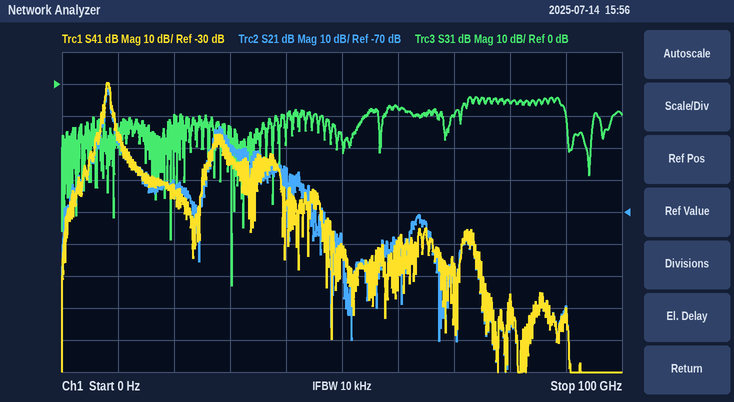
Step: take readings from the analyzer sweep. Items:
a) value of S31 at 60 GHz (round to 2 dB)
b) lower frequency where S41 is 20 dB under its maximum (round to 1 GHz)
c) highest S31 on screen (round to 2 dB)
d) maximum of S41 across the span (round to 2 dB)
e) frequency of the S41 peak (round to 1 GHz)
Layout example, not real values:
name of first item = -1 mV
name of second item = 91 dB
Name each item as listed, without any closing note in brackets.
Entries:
value of S31 at 60 GHz = -8 dB
lower frequency where S41 is 20 dB under its maximum = 6 GHz
highest S31 on screen = -4 dB
maximum of S41 across the span = -30 dB
frequency of the S41 peak = 8 GHz
